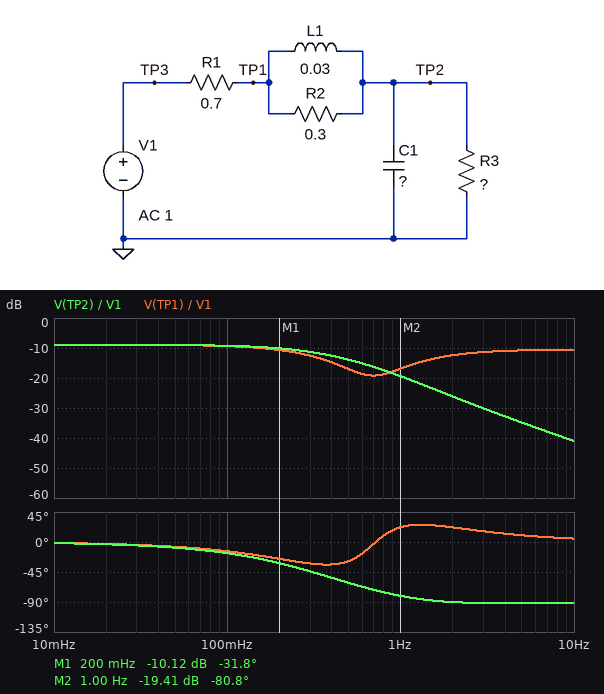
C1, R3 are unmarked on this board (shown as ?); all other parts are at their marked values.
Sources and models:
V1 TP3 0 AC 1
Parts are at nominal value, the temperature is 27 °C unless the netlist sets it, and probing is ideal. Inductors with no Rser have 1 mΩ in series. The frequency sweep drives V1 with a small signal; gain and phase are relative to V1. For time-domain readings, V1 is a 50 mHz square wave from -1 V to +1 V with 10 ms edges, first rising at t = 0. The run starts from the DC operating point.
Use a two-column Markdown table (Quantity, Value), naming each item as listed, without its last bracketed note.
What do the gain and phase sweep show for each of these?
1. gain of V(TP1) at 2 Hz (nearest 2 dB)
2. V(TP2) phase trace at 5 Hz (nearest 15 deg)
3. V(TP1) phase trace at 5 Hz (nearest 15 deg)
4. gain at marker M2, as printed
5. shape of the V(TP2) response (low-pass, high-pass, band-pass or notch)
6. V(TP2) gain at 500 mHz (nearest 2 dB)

| Quantity | Value |
|---|---|
| gain of V(TP1) at 2 Hz | -12 dB |
| V(TP2) phase trace at 5 Hz | -90 deg |
| V(TP1) phase trace at 5 Hz | 15 deg |
| gain at marker M2, as printed | -19.41 dB |
| shape of the V(TP2) response | low-pass |
| V(TP2) gain at 500 mHz | -14 dB |
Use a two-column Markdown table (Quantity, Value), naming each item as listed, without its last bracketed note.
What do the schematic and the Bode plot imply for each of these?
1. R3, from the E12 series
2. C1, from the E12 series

| Quantity | Value |
|---|---|
| R3, from the E12 series | 0.39 Ω |
| C1, from the E12 series | 1.8 F |
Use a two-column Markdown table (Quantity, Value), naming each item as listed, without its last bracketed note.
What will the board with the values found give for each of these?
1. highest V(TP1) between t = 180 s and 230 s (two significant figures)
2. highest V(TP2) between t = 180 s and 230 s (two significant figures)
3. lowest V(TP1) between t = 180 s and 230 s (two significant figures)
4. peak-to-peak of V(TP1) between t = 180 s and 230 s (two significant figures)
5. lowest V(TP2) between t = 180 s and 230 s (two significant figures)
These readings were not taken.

| Quantity | Value |
|---|---|
| highest V(TP1) between t = 180 s and 230 s | 360 mV |
| highest V(TP2) between t = 180 s and 230 s | 360 mV |
| lowest V(TP1) between t = 180 s and 230 s | -360 mV |
| peak-to-peak of V(TP1) between t = 180 s and 230 s | 720 mV |
| lowest V(TP2) between t = 180 s and 230 s | -360 mV |
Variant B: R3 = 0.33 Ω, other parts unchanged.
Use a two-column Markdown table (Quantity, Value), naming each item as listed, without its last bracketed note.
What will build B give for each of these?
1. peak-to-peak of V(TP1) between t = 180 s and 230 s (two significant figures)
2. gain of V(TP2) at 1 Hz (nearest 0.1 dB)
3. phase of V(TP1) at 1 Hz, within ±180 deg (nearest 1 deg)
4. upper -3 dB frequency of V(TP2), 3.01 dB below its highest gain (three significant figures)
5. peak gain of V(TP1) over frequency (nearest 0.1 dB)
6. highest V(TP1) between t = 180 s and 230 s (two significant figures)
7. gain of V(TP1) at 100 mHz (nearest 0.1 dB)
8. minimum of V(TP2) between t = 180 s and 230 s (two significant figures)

| Quantity | Value |
|---|---|
| peak-to-peak of V(TP1) between t = 180 s and 230 s | 640 mV |
| gain of V(TP2) at 1 Hz | -19.5 dB |
| phase of V(TP1) at 1 Hz, within ±180 deg | 22 deg |
| upper -3 dB frequency of V(TP2), 3.01 dB below its highest gain | 388 mHz |
| peak gain of V(TP1) over frequency | -9.9 dB |
| highest V(TP1) between t = 180 s and 230 s | 320 mV |
| gain of V(TP1) at 100 mHz | -10.3 dB |
| minimum of V(TP2) between t = 180 s and 230 s | -320 mV |
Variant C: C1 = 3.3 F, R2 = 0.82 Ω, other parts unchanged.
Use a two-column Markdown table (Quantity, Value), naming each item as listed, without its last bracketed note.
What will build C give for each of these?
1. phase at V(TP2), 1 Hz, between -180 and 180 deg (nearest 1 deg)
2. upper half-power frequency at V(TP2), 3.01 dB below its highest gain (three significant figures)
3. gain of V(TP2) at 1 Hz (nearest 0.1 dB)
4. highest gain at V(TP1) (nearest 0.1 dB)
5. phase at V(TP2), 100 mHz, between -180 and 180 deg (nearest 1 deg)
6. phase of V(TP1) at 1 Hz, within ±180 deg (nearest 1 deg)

| Quantity | Value |
|---|---|
| phase at V(TP2), 1 Hz, between -180 and 180 deg | -93 deg |
| upper half-power frequency at V(TP2), 3.01 dB below its highest gain | 195 mHz |
| gain of V(TP2) at 1 Hz | -24.0 dB |
| highest gain at V(TP1) | -5.4 dB |
| phase at V(TP2), 100 mHz, between -180 and 180 deg | -29 deg |
| phase of V(TP1) at 1 Hz, within ±180 deg | 60 deg |
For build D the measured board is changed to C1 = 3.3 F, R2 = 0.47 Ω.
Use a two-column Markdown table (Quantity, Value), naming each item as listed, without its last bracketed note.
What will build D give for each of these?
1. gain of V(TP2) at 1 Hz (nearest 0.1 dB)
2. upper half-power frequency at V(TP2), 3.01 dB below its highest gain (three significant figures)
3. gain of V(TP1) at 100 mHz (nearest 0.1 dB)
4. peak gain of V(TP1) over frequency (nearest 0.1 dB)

| Quantity | Value |
|---|---|
| gain of V(TP2) at 1 Hz | -24.2 dB |
| upper half-power frequency at V(TP2), 3.01 dB below its highest gain | 194 mHz |
| gain of V(TP1) at 100 mHz | -10.2 dB |
| peak gain of V(TP1) over frequency | -7.9 dB |
